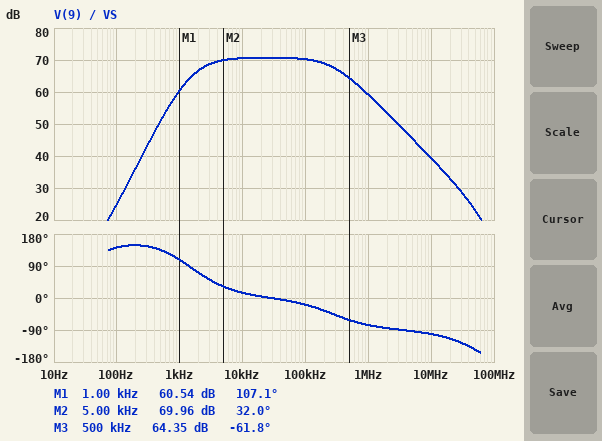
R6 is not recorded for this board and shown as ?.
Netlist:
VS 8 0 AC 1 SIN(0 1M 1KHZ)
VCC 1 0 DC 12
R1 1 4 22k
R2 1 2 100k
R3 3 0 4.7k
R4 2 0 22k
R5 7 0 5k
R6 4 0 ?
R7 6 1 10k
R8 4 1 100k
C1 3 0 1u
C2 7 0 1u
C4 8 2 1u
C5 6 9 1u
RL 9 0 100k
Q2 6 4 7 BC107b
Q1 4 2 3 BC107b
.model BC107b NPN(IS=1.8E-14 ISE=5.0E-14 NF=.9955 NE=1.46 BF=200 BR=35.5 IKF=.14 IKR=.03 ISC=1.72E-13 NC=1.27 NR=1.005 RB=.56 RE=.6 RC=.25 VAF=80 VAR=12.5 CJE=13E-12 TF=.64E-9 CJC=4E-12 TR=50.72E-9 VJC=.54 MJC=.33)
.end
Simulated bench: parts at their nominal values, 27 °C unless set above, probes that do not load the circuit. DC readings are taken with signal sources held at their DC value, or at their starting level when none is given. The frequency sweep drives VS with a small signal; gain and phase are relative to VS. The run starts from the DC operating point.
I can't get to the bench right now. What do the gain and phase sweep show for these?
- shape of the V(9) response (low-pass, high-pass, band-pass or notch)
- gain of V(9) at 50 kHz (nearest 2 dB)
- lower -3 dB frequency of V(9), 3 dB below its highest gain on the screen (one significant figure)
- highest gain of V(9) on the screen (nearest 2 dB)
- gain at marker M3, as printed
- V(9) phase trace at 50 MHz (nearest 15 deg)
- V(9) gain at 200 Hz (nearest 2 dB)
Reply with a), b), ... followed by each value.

a) band-pass
b) 70 dB
c) 2 kHz
d) 70 dB
e) 64.35 dB
f) -150 deg
g) 36 dB
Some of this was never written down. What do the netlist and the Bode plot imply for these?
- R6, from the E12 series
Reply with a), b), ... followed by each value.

a) 6.8 kΩ
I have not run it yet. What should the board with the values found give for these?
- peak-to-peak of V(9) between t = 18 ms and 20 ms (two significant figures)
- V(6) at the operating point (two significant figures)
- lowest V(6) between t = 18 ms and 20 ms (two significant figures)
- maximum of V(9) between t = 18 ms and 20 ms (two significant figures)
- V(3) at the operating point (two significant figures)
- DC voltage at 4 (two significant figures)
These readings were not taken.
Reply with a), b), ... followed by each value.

a) 2.1 V
b) 9.8 V
c) 8.7 V
d) 950 mV
e) 1.5 V
f) 1.7 V
